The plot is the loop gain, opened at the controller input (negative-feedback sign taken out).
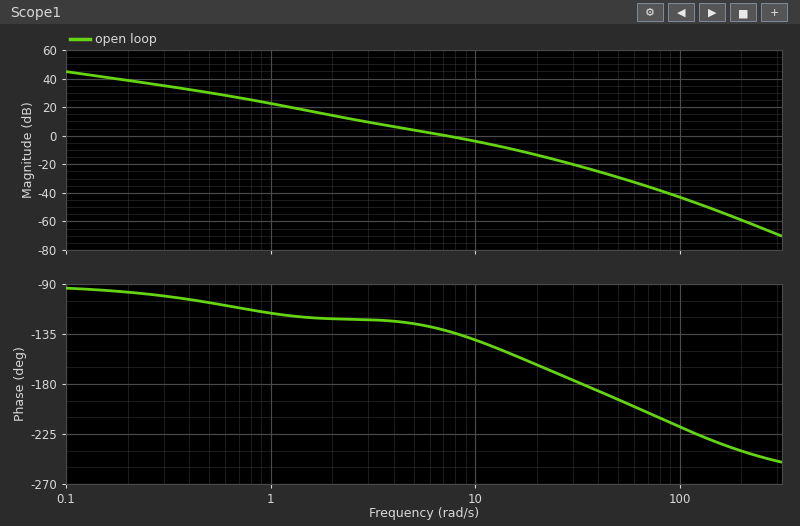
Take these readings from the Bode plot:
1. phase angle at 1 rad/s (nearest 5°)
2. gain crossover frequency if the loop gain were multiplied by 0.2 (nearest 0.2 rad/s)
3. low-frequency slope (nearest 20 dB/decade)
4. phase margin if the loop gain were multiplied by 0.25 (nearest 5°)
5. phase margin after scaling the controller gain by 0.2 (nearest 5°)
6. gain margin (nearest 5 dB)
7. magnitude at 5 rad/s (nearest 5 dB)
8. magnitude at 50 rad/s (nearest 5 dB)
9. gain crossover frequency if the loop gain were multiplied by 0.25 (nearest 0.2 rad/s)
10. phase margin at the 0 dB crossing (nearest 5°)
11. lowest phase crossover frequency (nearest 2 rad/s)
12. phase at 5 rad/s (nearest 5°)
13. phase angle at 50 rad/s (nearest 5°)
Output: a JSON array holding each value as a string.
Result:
["-115°", "2.0 rad/s", "-20 dB/decade", "60°", "60°", "20 dB", "5 dB", "-30 dB", "2.4 rad/s", "50°", "34 rad/s", "-125°", "-195°"]
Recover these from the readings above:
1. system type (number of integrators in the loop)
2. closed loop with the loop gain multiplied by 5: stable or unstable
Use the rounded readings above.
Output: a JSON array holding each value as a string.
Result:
["1", "stable"]
